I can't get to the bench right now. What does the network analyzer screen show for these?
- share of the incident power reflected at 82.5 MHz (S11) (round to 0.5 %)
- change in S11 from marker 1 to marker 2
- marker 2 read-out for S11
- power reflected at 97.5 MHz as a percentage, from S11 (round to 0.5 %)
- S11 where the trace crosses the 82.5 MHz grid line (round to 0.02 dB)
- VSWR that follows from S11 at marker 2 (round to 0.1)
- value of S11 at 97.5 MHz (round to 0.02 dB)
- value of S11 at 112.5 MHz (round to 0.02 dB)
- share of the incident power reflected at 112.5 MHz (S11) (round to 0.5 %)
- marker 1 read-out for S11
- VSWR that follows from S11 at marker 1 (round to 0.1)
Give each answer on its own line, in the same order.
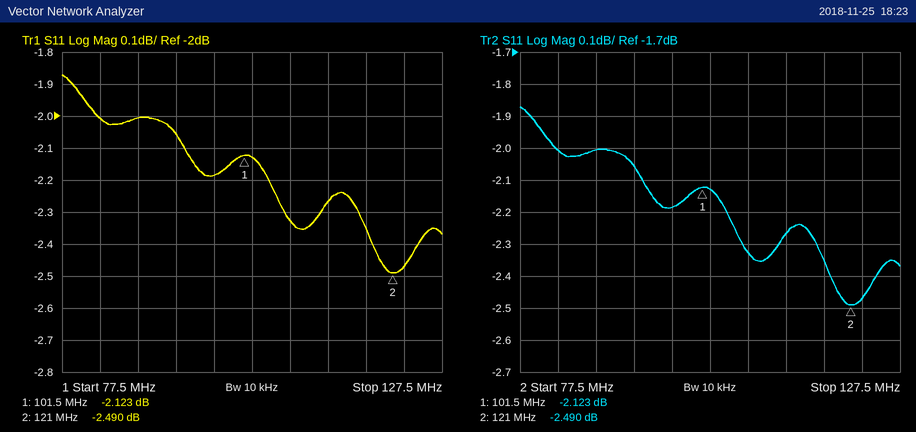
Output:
63.0 %
-0.367 dB
-2.490 dB
60.5 %
-2.00 dB
7.0
-2.18 dB
-2.26 dB
59.5 %
-2.123 dB
8.2
